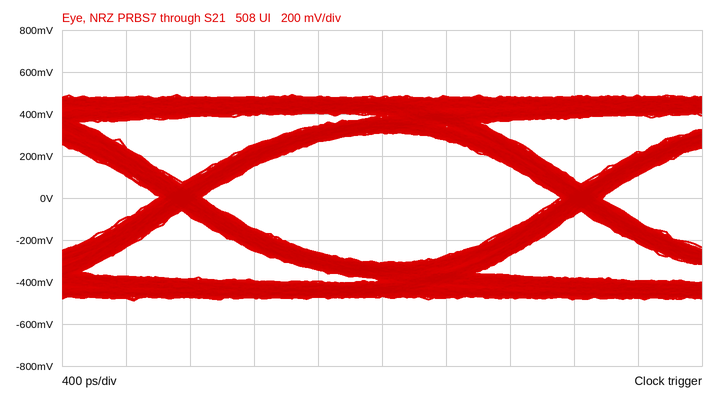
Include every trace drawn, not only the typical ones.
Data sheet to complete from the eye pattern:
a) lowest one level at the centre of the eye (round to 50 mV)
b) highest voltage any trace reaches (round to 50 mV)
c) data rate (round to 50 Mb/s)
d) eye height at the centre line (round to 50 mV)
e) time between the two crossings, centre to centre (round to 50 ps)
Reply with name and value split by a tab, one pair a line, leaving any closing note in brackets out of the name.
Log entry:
lowest one level at the centre of the eye	300 mV
highest voltage any trace reaches	500 mV
data rate	400 Mb/s
eye height at the centre line	600 mV
time between the two crossings, centre to centre	2.50 ns
